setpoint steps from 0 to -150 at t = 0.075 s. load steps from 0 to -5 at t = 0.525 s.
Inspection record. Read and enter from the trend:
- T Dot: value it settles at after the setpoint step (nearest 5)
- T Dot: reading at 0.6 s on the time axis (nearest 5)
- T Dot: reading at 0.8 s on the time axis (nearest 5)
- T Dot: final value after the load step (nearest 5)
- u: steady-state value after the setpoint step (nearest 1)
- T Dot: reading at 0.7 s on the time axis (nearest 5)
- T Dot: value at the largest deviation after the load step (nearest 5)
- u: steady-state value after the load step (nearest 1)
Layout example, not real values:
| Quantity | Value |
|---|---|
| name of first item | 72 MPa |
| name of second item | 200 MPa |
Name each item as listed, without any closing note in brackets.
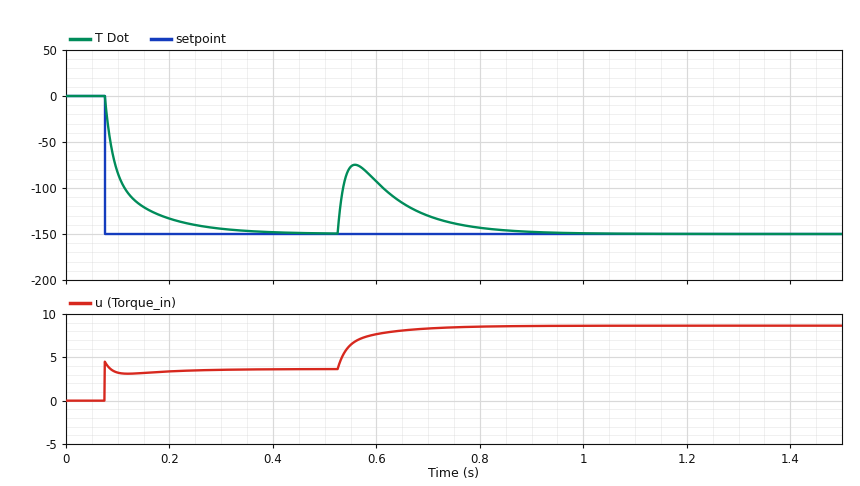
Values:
| Quantity | Value |
|---|---|
| T Dot: value it settles at after the setpoint step | -150 |
| T Dot: reading at 0.6 s on the time axis | -95 |
| T Dot: reading at 0.8 s on the time axis | -145 |
| T Dot: final value after the load step | -150 |
| u: steady-state value after the setpoint step | 4 |
| T Dot: reading at 0.7 s on the time axis | -130 |
| T Dot: value at the largest deviation after the load step | -75 |
| u: steady-state value after the load step | 9 |
